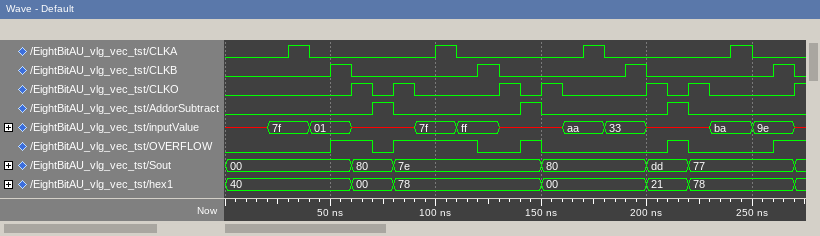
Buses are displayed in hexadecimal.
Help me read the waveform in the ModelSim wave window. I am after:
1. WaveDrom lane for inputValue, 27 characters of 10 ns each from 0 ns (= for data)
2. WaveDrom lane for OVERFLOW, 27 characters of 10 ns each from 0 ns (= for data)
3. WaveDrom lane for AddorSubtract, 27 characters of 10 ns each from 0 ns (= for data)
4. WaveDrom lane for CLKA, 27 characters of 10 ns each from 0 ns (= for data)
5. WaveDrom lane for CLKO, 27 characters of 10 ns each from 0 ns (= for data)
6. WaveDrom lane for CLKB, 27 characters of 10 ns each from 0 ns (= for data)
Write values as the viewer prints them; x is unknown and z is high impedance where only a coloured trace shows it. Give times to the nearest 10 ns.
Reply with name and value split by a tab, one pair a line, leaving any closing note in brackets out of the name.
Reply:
WaveDrom lane for inputValue, 27 characters of 10 ns each from 0 ns	{name: 'inputValue', wave: 'x.=.=.x..=.=.x..=.=.x..=.=.', data: '7f 01 7f ff aa 33 ba 9e'}
WaveDrom lane for OVERFLOW, 27 characters of 10 ns each from 0 ns	{name: 'OVERFLOW', wave: '0....1.01...0.10.....10...1'}
WaveDrom lane for AddorSubtract, 27 characters of 10 ns each from 0 ns	{name: 'AddorSubtract', wave: '0......10.....10.....10....'}
WaveDrom lane for CLKA, 27 characters of 10 ns each from 0 ns	{name: 'CLKA', wave: '0..10.....10.....10.....10.'}
WaveDrom lane for CLKO, 27 characters of 10 ns each from 0 ns	{name: 'CLKO', wave: '0.....1010...1010...1010...'}
WaveDrom lane for CLKB, 27 characters of 10 ns each from 0 ns	{name: 'CLKB', wave: '0....10.....10.....10.....1'}
